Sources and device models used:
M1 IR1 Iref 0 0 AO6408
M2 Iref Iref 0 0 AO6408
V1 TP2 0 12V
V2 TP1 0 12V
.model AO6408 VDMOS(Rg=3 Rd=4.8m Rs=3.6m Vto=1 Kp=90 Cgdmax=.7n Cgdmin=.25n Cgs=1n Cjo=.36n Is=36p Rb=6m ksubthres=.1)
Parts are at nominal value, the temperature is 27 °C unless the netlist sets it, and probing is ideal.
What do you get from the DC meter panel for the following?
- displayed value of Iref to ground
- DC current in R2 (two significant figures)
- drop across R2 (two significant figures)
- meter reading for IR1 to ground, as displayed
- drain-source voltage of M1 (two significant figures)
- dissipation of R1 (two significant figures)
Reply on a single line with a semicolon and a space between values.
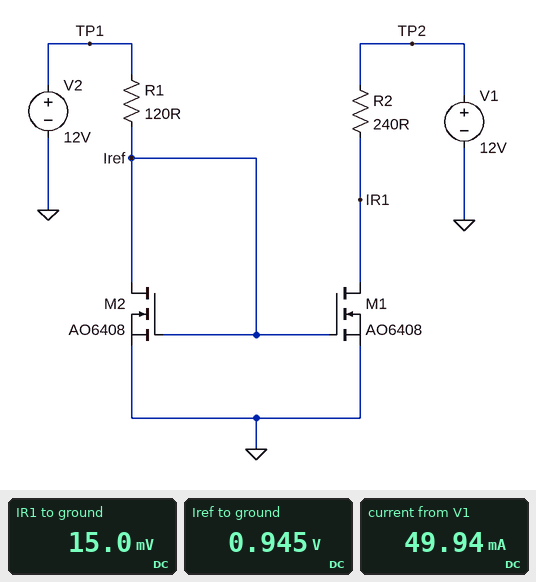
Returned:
0.945 V; 50 mA; 12 V; 15.0 mV; 15 mV; 1.0 W
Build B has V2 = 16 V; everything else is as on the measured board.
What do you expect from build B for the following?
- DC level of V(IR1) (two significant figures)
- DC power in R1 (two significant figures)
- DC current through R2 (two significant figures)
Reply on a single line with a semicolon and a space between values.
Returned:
12 mV; 1.9 W; 50 mA
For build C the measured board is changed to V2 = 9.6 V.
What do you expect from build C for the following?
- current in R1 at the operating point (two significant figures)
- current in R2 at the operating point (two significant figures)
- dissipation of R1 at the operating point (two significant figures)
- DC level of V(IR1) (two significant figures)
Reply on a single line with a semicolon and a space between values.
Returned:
72 mA; 50 mA; 630 mW; 18 mV
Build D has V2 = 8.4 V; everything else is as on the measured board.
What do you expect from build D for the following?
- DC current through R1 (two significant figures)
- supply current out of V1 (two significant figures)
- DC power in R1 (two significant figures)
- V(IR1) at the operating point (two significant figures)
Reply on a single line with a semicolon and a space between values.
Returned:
62 mA; 50 mA; 470 mW; 21 mV
